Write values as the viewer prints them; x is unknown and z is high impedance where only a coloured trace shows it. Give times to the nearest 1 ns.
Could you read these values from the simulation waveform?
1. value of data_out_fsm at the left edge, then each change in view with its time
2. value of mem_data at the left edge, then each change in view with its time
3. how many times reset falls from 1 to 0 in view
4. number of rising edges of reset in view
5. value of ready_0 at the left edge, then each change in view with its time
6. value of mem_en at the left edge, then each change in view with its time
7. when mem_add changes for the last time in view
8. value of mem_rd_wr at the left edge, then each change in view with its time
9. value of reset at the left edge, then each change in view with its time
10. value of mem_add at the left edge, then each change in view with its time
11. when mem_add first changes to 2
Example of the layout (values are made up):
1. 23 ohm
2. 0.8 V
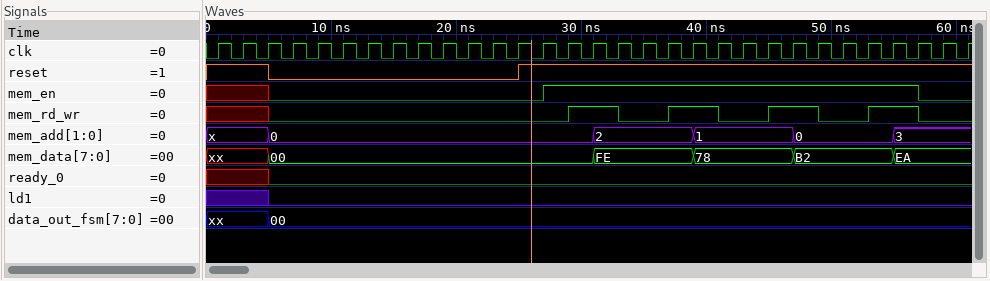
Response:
1. xx, 00 at 5 ns
2. xx, 00 at 5 ns, FE at 31 ns, 78 at 39 ns, B2 at 47 ns, EA at 55 ns
3. 1
4. 1
5. x, 0 at 5 ns
6. x, 0 at 5 ns, 1 at 27 ns, 0 at 57 ns
7. 55 ns
8. x, 0 at 5 ns, 1 at 29 ns, 0 at 33 ns, 1 at 37 ns, 0 at 41 ns, 1 at 45 ns, 0 at 49 ns, 1 at 53 ns, 0 at 57 ns
9. 1, 0 at 5 ns, 1 at 25 ns
10. x, 0 at 5 ns, 2 at 31 ns, 1 at 39 ns, 0 at 47 ns, 3 at 55 ns
11. 31 ns
